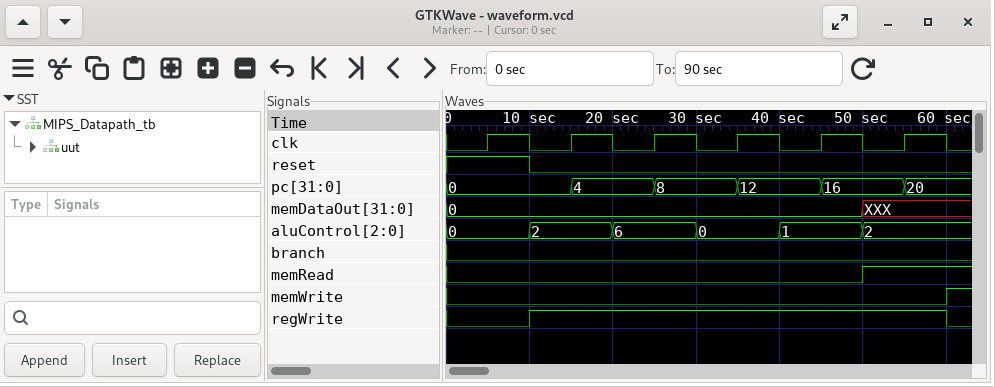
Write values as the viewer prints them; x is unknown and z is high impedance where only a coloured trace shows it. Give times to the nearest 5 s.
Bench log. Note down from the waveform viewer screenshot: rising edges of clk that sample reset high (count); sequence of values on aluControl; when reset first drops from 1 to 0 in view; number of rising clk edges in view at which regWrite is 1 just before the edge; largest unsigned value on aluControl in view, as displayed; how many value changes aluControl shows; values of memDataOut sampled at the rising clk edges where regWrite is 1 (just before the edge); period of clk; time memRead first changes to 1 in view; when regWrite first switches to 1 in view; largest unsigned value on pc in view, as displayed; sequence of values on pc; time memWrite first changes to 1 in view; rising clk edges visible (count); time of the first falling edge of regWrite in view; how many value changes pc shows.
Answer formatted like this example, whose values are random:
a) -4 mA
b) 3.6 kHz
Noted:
a) 1
b) 0, 2, 6, 0, 1, 2
c) 10 s
d) 5
e) 6
f) 5
g) 0, 0, 0, 0, XXX
h) 10 s
i) 50 s
j) 10 s
k) 20
l) 0, 4, 8, 12, 16, 20
m) 60 s
n) 6
o) 60 s
p) 5
